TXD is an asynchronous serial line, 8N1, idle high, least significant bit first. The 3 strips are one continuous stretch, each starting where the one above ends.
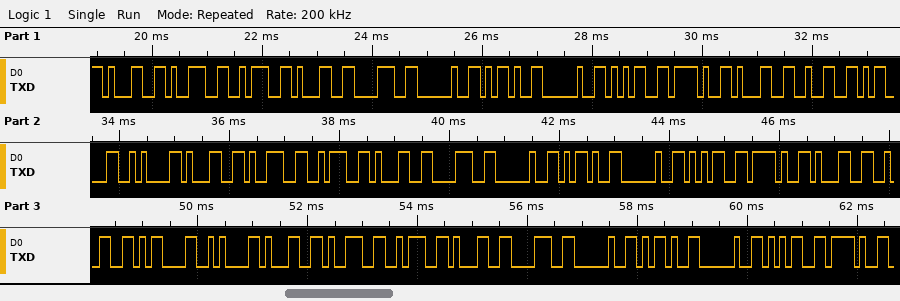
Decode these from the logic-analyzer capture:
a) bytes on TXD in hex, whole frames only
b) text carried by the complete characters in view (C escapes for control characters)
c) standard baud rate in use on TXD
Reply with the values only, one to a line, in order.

31 39 3A 31 38 20 2D 20 35 2F 31 32 0D 0A 31 39 3A 31 38 20 2D 20 35 2F 31 32 0D 0A 31 39 3A 31 38 20 2D 20 35 2F
"19:18 - 5/12\r\n19:18 - 5/12\r\n19:18 - 5/"
9600 baud
